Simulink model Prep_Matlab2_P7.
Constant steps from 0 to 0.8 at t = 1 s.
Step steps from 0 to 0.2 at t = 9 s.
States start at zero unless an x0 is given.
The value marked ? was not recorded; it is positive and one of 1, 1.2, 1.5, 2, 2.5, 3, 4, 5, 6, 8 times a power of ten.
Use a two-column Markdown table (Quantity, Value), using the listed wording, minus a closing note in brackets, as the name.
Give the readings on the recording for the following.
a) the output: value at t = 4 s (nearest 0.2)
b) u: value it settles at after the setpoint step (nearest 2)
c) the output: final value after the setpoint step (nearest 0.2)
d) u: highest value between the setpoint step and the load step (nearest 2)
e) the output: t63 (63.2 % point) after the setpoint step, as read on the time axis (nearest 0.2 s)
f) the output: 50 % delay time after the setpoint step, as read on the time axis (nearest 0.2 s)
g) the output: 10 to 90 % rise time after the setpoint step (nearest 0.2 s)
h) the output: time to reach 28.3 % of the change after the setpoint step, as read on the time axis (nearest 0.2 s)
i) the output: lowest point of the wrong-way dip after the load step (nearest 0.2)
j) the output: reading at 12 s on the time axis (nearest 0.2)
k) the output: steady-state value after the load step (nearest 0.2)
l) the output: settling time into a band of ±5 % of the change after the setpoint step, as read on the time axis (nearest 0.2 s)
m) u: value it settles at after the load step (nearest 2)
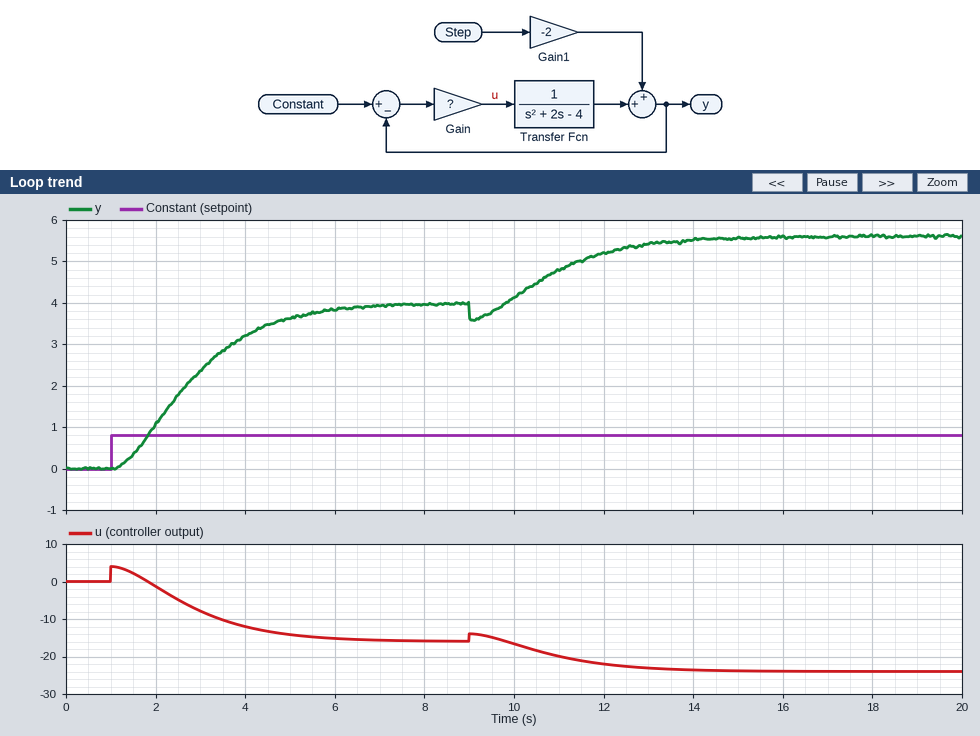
| Quantity | Value |
|---|---|
| the output: value at t = 4 s | 3.2 |
| u: value it settles at after the setpoint step | -16 |
| the output: final value after the setpoint step | 4.0 |
| u: highest value between the setpoint step and the load step | 4 |
| the output: t63 (63.2 % point) after the setpoint step, as read on the time axis | 3.2 s |
| the output: 50 % delay time after the setpoint step, as read on the time axis | 2.6 s |
| the output: 10 to 90 % rise time after the setpoint step | 3.4 s |
| the output: time to reach 28.3 % of the change after the setpoint step, as read on the time axis | 2.0 s |
| the output: lowest point of the wrong-way dip after the load step | 3.6 |
| the output: reading at 12 s on the time axis | 5.2 |
| the output: steady-state value after the load step | 5.6 |
| the output: settling time into a band of ±5 % of the change after the setpoint step, as read on the time axis | 5.8 s |
| u: value it settles at after the load step | -24 |
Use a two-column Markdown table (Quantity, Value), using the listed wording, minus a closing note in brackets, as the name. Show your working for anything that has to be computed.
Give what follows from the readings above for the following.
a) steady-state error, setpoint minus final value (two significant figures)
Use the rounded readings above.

| Quantity | Value |
|---|---|
| steady-state error, setpoint minus final value | 0.8 - 4 = -3.2 |
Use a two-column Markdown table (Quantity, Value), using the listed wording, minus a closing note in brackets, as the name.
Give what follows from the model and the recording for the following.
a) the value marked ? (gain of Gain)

| Quantity | Value |
|---|---|
| the value marked ? | 5 |
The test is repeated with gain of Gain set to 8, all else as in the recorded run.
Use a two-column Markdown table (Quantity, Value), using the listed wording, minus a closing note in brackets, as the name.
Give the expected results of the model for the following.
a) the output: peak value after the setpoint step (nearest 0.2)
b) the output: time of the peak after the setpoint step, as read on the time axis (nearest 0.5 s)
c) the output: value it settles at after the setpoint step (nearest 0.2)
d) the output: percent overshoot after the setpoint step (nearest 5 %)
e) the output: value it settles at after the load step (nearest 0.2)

| Quantity | Value |
|---|---|
| the output: peak value after the setpoint step | 1.8 |
| the output: time of the peak after the setpoint step, as read on the time axis | 3.0 s |
| the output: value it settles at after the setpoint step | 1.6 |
| the output: percent overshoot after the setpoint step | 15 % |
| the output: value it settles at after the load step | 2.0 |
